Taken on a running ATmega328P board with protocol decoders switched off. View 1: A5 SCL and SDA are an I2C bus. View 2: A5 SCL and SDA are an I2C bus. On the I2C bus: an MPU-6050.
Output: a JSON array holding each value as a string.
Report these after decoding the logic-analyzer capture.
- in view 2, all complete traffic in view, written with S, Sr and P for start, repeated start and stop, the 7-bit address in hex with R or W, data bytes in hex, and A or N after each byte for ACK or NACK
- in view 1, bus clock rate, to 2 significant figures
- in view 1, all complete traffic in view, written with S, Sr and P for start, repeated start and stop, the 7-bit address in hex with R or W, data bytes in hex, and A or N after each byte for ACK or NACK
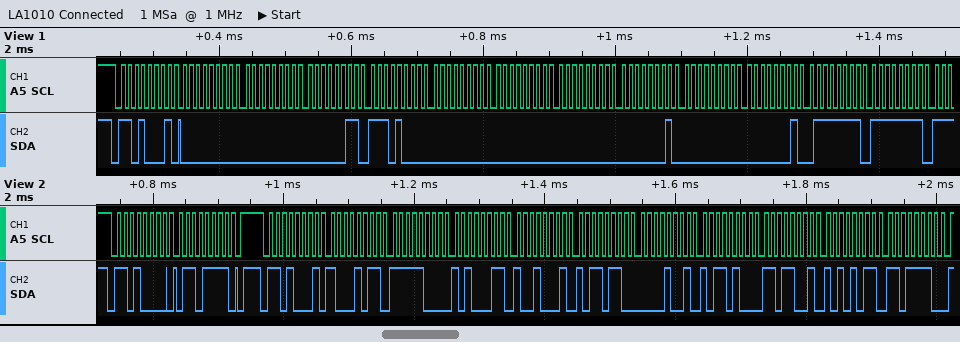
["S 68W A 6F A P S 68R A 8B A F8 A A3 A 91 A B6 A 09 A B4 A D9 A AB A DE A", "100 kHz", "S 68R A 00 A 00 A 03 A E8 A 00 A 00 A 00 A 01 A 00 A 01 A 7F A FF A"]
